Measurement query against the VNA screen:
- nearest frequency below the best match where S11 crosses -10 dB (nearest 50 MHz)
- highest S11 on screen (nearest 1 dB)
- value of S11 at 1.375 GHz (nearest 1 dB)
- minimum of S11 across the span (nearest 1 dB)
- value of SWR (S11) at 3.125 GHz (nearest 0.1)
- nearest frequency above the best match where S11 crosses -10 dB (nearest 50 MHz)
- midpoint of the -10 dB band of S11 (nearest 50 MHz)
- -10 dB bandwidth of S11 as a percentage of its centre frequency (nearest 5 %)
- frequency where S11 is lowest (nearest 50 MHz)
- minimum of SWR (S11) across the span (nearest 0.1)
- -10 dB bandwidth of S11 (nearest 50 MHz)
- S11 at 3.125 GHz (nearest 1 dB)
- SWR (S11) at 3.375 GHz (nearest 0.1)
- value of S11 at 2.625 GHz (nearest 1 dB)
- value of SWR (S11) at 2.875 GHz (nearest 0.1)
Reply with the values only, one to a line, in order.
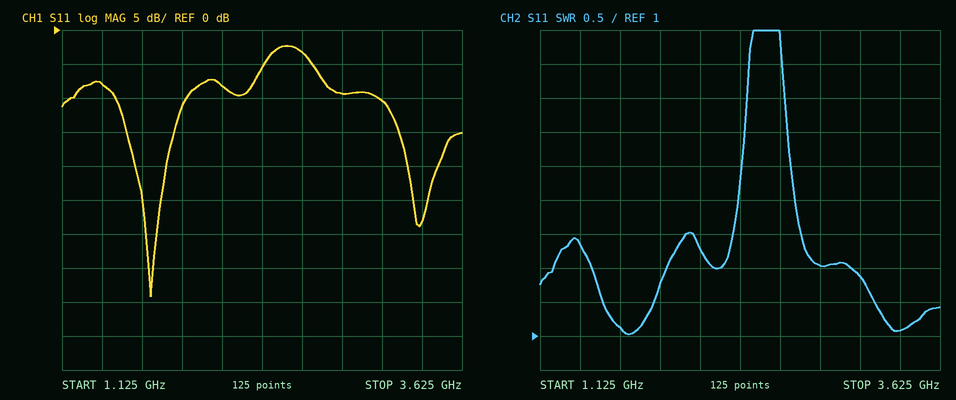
1.45 GHz
-2 dB
-8 dB
-39 dB
1.9
1.90 GHz
1.70 GHz
25 %
1.70 GHz
1.0
450 MHz
-10 dB
1.1
-3 dB
2.0
